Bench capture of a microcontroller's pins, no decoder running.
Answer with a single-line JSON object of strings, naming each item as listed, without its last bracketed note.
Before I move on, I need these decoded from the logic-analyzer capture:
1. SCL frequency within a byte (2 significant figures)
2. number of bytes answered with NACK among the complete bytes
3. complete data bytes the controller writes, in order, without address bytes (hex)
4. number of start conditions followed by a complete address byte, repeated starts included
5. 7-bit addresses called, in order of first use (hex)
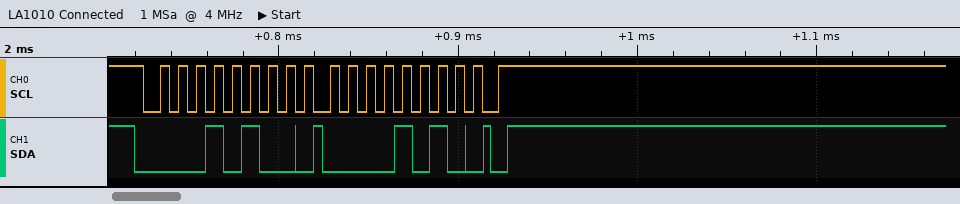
{"SCL frequency within a byte": "100 kHz", "number of bytes answered with NACK among the complete bytes": "0", "complete data bytes the controller writes, in order, without address bytes": "0A", "number of start conditions followed by a complete address byte, repeated starts included": "1", "7-bit addresses called, in order of first use": "0x0A"}
